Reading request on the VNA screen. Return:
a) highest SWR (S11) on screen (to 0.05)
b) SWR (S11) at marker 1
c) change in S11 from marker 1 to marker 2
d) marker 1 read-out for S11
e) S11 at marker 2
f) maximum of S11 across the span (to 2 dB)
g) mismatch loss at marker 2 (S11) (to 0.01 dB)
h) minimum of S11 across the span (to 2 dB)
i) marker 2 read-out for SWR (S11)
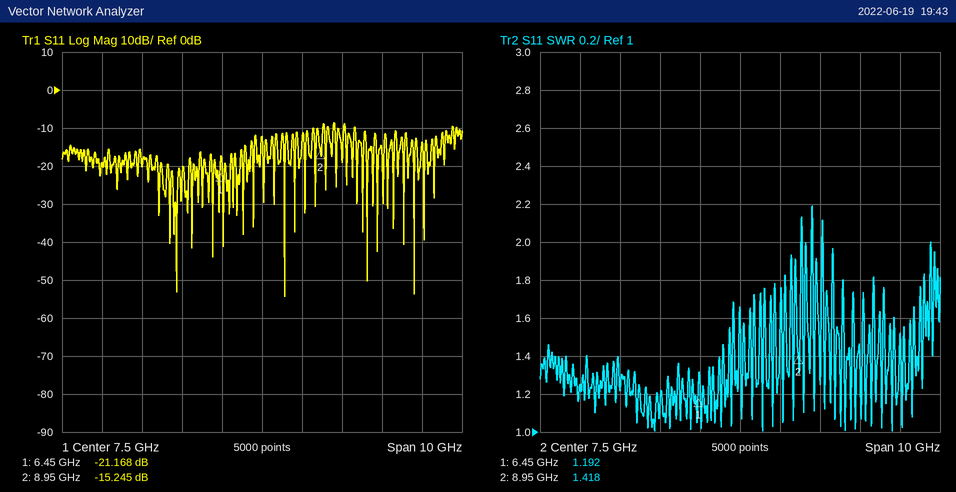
2.20
1.192
5.923 dB
-21.168 dB
-15.245 dB
-8 dB
0.13 dB
-54 dB
1.418
